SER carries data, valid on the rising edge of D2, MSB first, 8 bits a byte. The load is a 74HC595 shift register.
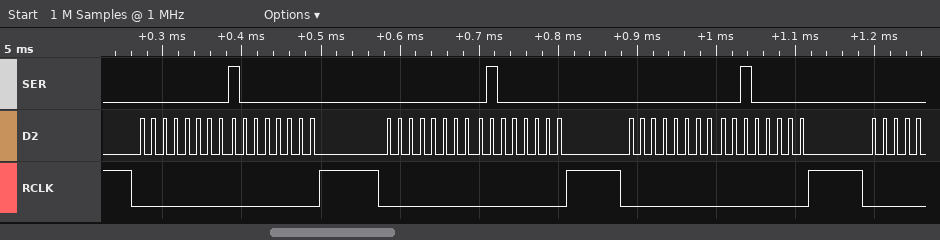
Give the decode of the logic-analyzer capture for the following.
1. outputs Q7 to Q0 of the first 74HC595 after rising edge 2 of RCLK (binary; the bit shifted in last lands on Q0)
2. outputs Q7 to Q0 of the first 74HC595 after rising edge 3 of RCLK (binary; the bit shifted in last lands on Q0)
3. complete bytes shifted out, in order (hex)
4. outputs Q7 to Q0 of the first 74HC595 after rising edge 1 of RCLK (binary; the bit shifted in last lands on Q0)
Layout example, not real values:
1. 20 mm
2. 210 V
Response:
1. 01000000
2. 00100000
3. 00 80 00 40 00 20
4. 10000000
